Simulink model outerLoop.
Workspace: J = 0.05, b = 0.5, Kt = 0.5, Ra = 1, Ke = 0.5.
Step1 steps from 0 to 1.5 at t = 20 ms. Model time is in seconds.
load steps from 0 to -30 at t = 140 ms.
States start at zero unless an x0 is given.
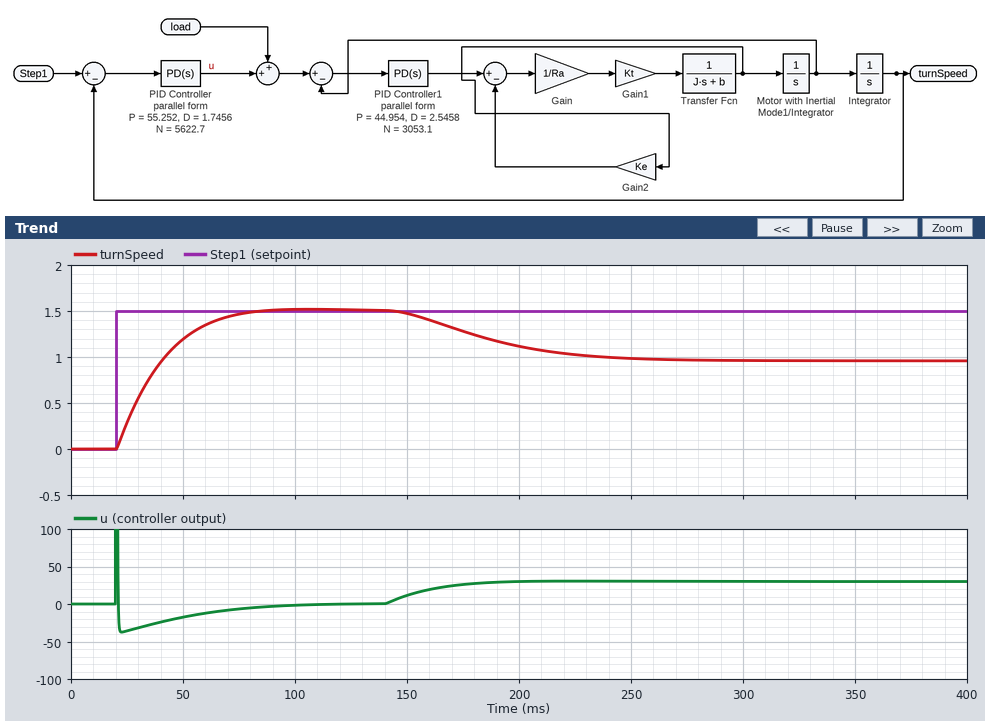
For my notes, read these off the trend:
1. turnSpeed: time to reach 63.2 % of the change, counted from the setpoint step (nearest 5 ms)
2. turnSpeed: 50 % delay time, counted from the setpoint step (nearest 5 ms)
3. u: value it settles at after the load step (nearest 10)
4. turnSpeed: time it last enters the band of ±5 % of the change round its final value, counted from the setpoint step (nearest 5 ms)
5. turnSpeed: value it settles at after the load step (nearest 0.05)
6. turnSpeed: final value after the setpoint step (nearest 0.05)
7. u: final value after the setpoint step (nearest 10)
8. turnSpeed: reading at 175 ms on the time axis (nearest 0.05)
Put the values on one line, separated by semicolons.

20 ms; 15 ms; 30; 50 ms; 0.95; 1.50; 0; 1.30
